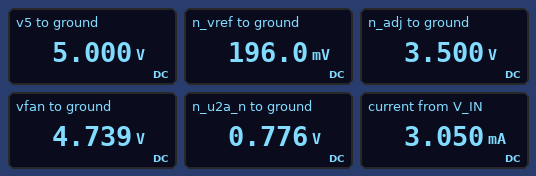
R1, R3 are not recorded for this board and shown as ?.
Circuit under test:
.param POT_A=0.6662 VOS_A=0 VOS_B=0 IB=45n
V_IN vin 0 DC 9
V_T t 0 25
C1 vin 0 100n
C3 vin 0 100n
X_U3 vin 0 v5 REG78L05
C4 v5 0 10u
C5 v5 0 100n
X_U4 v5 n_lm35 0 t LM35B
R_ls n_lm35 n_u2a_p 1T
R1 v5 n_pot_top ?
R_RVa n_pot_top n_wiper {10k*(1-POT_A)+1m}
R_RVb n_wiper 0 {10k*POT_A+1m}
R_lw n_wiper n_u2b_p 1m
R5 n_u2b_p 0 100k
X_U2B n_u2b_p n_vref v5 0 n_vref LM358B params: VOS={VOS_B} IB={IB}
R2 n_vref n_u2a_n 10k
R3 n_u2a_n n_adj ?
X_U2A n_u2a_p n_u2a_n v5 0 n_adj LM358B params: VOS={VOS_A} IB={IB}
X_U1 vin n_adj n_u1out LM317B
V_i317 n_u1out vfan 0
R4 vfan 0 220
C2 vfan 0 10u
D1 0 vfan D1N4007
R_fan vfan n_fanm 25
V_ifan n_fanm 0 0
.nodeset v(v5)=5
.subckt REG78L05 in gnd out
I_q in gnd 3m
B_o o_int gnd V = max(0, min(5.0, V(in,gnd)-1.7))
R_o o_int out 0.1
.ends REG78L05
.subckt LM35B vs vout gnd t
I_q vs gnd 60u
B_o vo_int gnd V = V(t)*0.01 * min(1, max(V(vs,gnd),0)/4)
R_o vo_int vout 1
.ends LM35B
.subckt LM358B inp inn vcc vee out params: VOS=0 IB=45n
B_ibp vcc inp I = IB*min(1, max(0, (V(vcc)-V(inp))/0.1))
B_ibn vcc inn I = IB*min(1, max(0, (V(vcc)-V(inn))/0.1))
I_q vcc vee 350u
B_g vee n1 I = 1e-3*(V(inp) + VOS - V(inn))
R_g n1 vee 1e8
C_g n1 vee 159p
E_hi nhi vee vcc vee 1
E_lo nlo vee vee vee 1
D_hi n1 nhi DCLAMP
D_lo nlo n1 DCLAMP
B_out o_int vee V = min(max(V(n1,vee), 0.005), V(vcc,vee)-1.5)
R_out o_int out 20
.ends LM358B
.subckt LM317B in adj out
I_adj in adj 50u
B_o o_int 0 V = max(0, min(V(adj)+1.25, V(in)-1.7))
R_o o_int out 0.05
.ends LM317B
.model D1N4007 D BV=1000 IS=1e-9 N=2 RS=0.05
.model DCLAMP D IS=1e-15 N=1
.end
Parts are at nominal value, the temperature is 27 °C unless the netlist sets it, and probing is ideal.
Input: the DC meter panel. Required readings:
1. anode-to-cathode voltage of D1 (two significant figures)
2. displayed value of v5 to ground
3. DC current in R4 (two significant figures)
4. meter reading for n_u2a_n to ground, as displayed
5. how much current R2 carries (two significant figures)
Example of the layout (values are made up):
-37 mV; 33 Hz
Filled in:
-4.7 V; 5.000 V; 22 mA; 0.776 V; 58 µA
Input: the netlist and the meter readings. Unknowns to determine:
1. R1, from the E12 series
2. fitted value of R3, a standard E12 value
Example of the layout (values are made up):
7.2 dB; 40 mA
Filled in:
150 kΩ; 47 kΩ
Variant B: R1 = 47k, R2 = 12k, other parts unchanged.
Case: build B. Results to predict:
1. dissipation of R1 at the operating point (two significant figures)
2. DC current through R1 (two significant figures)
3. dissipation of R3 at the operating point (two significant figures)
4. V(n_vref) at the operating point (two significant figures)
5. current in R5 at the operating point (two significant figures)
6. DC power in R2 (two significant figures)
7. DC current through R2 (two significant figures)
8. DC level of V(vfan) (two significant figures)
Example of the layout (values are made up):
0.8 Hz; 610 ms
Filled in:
370 µW; 88 µA; 120 µW; 550 mV; 5.5 µA; 30 µW; 50 µA; 4.7 V
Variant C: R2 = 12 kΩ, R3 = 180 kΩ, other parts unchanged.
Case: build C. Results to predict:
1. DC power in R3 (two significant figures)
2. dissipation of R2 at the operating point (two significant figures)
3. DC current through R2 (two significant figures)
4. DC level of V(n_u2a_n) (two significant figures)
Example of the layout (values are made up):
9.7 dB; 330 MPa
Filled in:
53 µW; 3.6 µW; 17 µA; 400 mV
